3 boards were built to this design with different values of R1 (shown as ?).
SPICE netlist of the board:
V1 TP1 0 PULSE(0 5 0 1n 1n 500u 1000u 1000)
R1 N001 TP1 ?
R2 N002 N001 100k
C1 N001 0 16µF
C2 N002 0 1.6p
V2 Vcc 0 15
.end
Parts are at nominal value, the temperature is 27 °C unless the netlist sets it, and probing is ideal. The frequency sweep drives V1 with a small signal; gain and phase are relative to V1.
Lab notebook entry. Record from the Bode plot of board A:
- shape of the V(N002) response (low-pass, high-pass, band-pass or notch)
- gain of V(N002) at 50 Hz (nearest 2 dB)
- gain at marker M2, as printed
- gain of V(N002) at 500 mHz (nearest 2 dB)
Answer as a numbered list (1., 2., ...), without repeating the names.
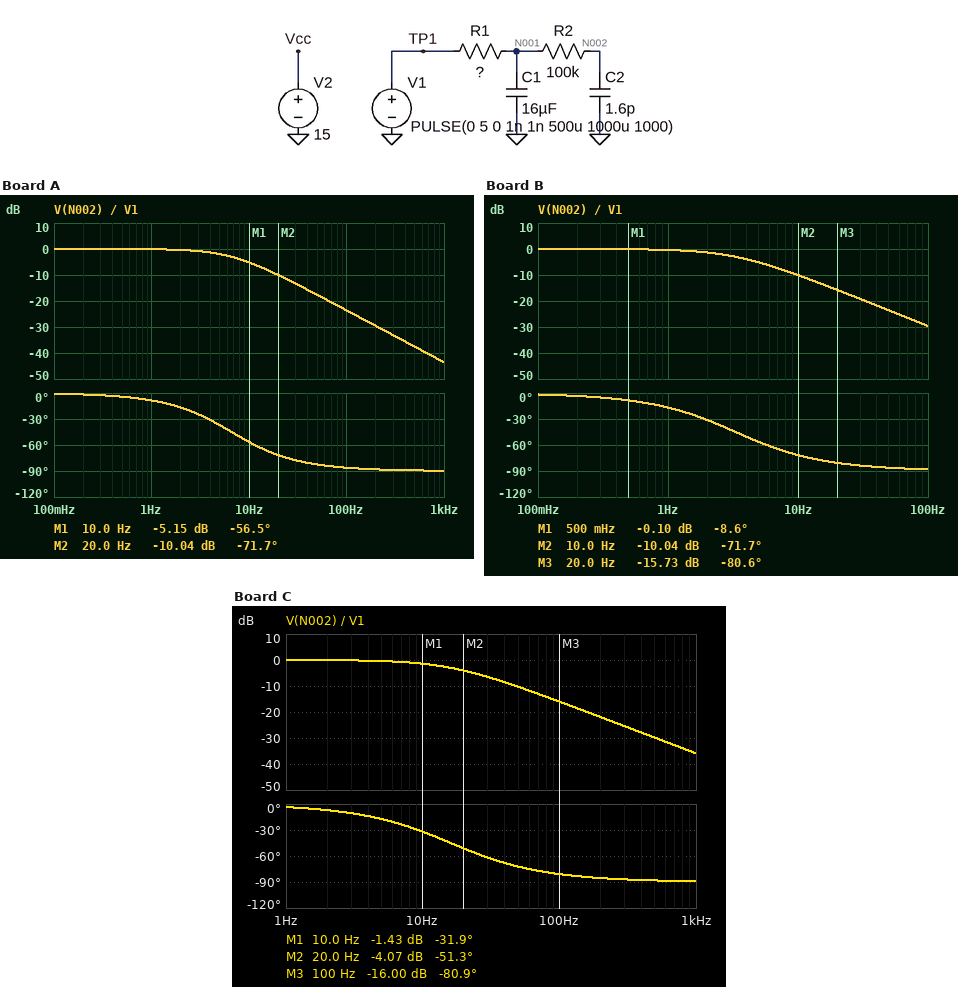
1. low-pass
2. -18 dB
3. -10.04 dB
4. 0 dB
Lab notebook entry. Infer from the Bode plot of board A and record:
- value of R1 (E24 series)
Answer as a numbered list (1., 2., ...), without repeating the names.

1. 1.5 kΩ
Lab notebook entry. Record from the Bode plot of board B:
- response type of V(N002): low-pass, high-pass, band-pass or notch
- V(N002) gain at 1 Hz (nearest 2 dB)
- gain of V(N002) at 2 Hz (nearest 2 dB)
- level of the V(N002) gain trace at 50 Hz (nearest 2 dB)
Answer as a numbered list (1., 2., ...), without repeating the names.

1. low-pass
2. 0 dB
3. -2 dB
4. -24 dB
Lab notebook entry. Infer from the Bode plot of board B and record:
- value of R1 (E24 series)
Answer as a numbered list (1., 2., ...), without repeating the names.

1. 3 kΩ
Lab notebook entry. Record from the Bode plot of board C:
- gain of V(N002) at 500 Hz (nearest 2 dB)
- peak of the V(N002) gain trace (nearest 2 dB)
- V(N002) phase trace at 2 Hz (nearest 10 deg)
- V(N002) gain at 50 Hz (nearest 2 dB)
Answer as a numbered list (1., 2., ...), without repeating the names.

1. -30 dB
2. 0 dB
3. -10 deg
4. -10 dB
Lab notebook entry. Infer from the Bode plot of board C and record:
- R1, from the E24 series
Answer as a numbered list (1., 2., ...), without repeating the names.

1. 620 Ω
